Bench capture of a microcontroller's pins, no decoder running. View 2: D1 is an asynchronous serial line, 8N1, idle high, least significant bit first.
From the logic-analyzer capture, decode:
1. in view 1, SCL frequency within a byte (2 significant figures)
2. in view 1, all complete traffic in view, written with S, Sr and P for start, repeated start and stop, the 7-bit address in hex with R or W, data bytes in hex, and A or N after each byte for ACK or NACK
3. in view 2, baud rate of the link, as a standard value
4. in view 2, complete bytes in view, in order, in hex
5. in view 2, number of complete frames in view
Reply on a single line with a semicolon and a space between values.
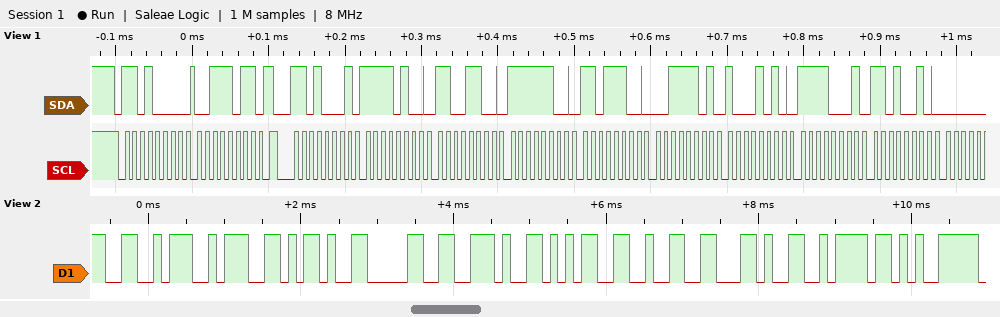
100 kHz; S 68W A 3B A Sr 68R A F4 A CC A FC A DC A 3D A 8A A F1 A D2 A; 9600 baud; A6 3A 2D 30 2E 35 32 2C 7A E5; 10
